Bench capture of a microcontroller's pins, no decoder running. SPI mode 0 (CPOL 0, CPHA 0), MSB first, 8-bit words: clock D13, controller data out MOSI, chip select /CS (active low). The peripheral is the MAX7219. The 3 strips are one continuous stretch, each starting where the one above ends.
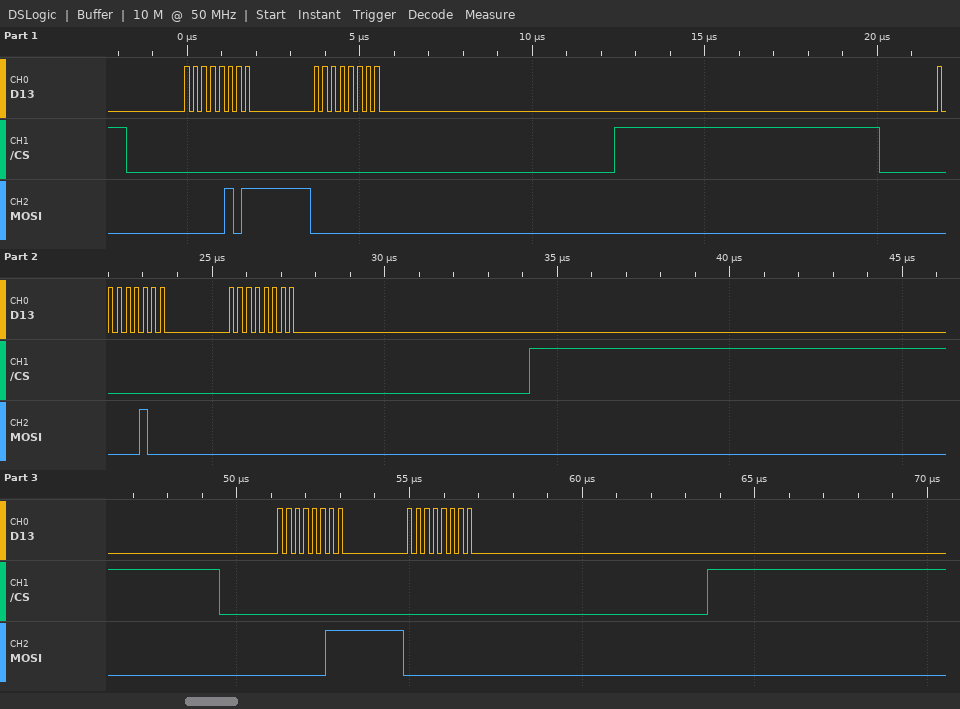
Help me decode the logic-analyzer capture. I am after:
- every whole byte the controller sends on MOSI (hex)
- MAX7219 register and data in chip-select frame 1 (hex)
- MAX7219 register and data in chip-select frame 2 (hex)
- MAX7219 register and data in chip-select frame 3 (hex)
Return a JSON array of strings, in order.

["05 00 04 00 03 00", "register 0x5, data 0x00", "register 0x4, data 0x00", "register 0x3, data 0x00"]
